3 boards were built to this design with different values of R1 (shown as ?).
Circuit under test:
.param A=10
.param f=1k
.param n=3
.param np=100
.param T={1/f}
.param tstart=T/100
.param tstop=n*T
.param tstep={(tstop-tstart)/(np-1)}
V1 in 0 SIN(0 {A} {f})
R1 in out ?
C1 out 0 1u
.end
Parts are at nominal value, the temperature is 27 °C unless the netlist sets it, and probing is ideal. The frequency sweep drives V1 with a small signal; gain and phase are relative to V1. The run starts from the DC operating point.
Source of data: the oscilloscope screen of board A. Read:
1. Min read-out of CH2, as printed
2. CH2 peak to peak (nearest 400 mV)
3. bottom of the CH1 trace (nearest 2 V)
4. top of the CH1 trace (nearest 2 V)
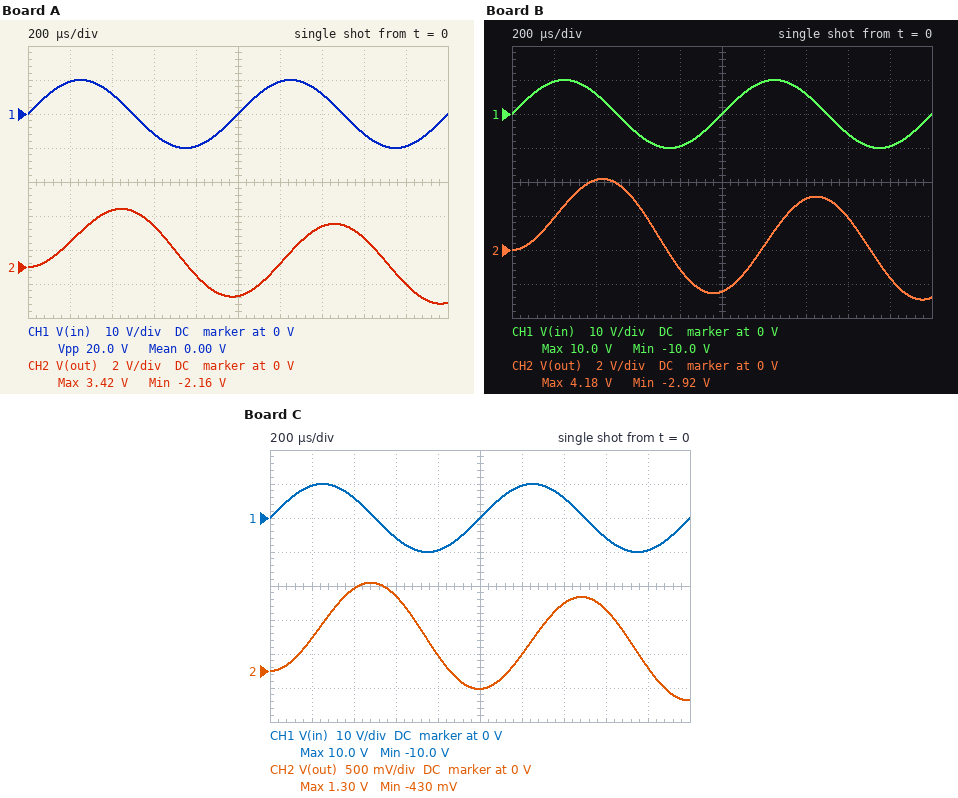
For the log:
-2.16 V
5.6 V
-10 V
10 V
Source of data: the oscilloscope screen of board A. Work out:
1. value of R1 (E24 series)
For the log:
680 Ω
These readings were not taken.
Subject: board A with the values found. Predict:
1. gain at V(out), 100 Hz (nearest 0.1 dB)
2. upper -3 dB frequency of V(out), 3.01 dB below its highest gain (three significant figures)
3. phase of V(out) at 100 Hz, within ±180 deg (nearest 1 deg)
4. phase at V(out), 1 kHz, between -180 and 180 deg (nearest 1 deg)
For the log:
-0.7 dB
234 Hz
-23 deg
-77 deg
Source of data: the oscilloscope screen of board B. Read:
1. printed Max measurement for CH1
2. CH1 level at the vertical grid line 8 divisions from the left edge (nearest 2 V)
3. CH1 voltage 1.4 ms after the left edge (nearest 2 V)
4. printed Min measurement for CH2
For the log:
10.0 V
-6 V
6 V
-2.92 V
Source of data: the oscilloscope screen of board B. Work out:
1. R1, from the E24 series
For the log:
510 Ω
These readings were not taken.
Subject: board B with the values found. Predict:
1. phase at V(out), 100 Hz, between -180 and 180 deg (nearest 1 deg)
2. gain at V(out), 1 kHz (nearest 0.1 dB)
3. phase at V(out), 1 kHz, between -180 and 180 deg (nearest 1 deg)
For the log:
-18 deg
-10.5 dB
-73 deg
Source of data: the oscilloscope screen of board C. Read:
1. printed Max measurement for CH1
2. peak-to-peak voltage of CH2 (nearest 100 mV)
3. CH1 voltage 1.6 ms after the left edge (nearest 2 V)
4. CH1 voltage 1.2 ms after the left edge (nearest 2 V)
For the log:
10.0 V
1.7 V
-6 V
10 V
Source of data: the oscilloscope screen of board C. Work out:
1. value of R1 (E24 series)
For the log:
2.2 kΩ
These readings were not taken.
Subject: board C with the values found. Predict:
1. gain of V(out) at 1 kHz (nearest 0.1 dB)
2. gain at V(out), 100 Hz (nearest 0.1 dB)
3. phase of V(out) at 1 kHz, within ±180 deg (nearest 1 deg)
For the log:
-22.8 dB
-4.6 dB
-86 deg
